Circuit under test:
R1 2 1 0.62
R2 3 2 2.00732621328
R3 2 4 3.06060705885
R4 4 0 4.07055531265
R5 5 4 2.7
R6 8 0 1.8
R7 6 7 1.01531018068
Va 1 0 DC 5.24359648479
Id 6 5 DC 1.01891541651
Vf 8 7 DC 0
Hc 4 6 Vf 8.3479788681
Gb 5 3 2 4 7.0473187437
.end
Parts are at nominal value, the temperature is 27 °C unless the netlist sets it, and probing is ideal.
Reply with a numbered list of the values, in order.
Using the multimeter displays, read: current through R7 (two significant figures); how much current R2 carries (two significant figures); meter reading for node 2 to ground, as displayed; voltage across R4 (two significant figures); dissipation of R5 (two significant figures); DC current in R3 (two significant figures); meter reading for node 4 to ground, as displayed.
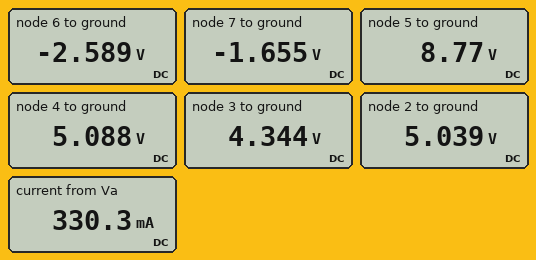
1. 920 mA
2. 350 mA
3. 5.039 V
4. 5.1 V
5. 5.0 W
6. 16 mA
7. 5.088 V
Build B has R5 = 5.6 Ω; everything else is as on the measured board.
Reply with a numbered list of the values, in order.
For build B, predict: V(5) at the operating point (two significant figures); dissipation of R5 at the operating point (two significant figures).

1. 13 V
2. 10 W
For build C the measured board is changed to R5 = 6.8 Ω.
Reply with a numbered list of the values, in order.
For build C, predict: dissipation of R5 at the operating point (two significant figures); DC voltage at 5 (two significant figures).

1. 13 W
2. 14 V
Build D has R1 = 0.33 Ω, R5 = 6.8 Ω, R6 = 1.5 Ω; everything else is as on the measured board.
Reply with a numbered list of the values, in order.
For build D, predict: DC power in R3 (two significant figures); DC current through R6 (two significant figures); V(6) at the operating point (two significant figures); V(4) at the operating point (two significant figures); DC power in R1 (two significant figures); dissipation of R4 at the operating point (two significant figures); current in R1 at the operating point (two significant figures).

1. 1.1 mW
2. 890 mA
3. -2.2 V
4. 5.2 V
5. 49 mW
6. 6.6 W
7. 380 mA
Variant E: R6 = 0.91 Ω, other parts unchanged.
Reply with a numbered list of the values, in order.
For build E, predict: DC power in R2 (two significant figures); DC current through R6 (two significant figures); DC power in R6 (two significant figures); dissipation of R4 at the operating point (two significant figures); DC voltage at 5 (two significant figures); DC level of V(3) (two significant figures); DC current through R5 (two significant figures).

1. 450 mW
2. 780 mA
3. 560 mW
4. 6.2 W
5. 9.1 V
6. 4.0 V
7. 1.5 A
